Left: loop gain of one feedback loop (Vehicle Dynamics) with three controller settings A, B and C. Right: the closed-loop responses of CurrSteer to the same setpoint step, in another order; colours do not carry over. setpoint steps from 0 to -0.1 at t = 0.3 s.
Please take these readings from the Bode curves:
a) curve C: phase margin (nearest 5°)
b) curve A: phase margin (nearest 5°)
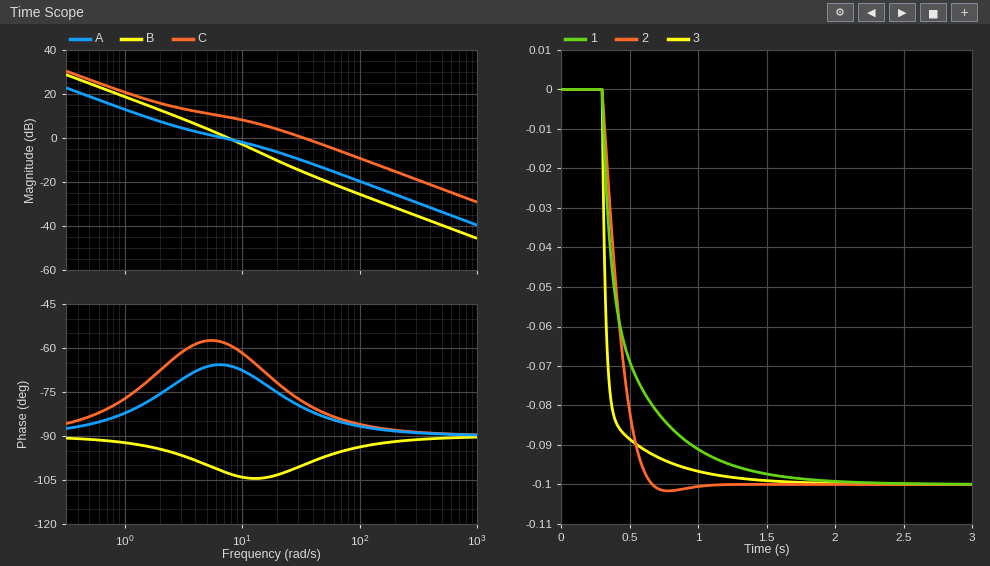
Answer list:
100°
115°
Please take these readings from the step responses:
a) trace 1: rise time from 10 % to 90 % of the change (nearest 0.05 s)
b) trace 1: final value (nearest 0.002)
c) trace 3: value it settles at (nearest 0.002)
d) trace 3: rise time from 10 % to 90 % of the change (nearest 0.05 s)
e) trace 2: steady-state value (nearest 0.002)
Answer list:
0.65 s
-0.100
-0.100
0.25 s
-0.100
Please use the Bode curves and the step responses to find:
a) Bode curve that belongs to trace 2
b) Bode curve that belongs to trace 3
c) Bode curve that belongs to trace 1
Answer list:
B
C
A
